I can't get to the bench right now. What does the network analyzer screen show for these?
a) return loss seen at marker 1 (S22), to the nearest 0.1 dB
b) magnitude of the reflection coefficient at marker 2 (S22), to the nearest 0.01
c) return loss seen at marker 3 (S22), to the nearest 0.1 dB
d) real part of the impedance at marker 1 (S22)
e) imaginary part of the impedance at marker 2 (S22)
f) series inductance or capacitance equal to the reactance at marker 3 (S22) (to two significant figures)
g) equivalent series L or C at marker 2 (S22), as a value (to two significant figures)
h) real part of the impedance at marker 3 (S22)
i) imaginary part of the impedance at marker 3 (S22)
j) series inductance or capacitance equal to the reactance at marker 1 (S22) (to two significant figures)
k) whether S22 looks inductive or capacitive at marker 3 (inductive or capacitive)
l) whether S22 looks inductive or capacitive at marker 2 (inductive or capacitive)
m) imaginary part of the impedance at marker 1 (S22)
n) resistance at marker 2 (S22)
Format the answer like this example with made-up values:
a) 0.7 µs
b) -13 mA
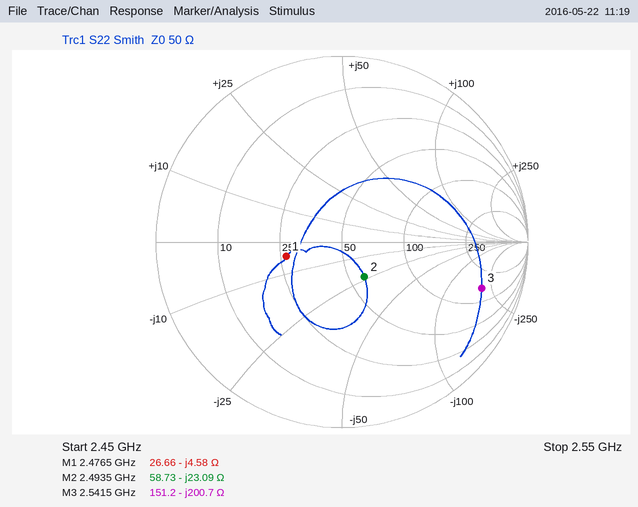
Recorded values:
a) 10.2 dB
b) 0.22
c) 2.0 dB
d) 26.66 Ω
e) -23.09 Ω
f) 310 fF
g) 2.8 pF
h) 151.2 Ω
i) -200.7 Ω
j) 14 pF
k) capacitive
l) capacitive
m) -4.58 Ω
n) 58.73 Ω
